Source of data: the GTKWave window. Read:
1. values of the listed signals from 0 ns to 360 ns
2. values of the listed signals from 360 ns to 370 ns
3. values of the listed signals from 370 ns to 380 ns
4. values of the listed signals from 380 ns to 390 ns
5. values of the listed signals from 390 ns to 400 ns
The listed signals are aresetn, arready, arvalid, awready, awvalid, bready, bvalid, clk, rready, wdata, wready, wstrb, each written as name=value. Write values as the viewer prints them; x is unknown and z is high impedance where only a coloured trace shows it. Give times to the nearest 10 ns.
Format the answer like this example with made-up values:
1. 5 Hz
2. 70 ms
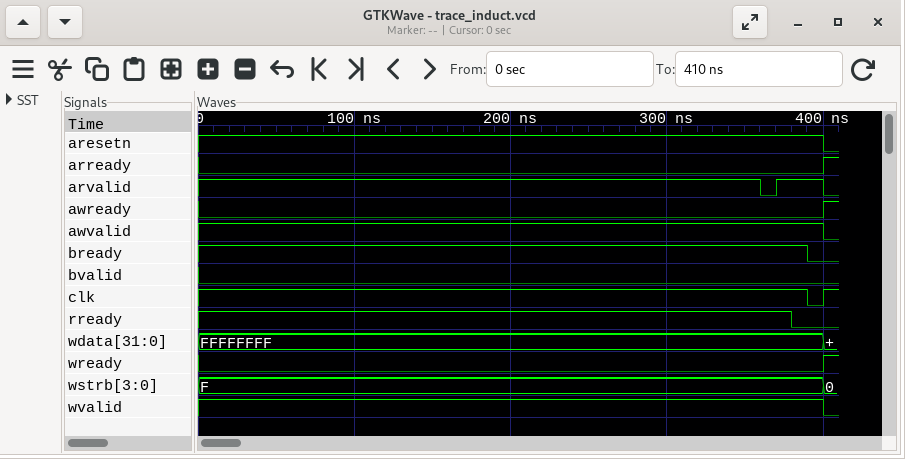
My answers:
1. aresetn=1, arready=0, arvalid=1, awready=0, awvalid=1, bready=1, bvalid=0, clk=1, rready=1, wdata=FFFFFFFF, wready=0, wstrb=F
2. aresetn=1, arready=0, arvalid=0, awready=0, awvalid=1, bready=1, bvalid=0, clk=1, rready=1, wdata=FFFFFFFF, wready=0, wstrb=F
3. aresetn=1, arready=0, arvalid=1, awready=0, awvalid=1, bready=1, bvalid=0, clk=1, rready=1, wdata=FFFFFFFF, wready=0, wstrb=F
4. aresetn=1, arready=0, arvalid=1, awready=0, awvalid=1, bready=1, bvalid=0, clk=1, rready=0, wdata=FFFFFFFF, wready=0, wstrb=F
5. aresetn=1, arready=0, arvalid=1, awready=0, awvalid=1, bready=0, bvalid=0, clk=0, rready=0, wdata=FFFFFFFF, wready=0, wstrb=F
